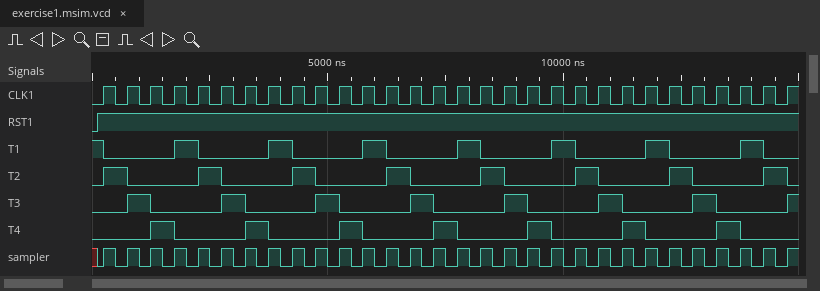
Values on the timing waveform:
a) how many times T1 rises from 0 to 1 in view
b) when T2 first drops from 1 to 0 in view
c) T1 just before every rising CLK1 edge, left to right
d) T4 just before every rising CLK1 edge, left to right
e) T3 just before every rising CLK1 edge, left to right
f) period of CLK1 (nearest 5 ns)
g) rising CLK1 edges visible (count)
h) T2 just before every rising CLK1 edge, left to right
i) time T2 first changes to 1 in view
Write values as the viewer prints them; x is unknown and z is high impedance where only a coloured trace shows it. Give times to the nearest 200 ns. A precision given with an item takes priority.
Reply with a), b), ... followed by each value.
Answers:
a) 7
b) 800 ns
c) 1 0 0 0 1 0 0 0 1 0 0 0 1 0 0 0 1 0 0 0 1 0 0 0 1 0 0 0 1 0
d) 0 0 0 1 0 0 0 1 0 0 0 1 0 0 0 1 0 0 0 1 0 0 0 1 0 0 0 1 0 0
e) 0 0 1 0 0 0 1 0 0 0 1 0 0 0 1 0 0 0 1 0 0 0 1 0 0 0 1 0 0 0
f) 500 ns
g) 30
h) 0 1 0 0 0 1 0 0 0 1 0 0 0 1 0 0 0 1 0 0 0 1 0 0 0 1 0 0 0 1
i) 200 ns
